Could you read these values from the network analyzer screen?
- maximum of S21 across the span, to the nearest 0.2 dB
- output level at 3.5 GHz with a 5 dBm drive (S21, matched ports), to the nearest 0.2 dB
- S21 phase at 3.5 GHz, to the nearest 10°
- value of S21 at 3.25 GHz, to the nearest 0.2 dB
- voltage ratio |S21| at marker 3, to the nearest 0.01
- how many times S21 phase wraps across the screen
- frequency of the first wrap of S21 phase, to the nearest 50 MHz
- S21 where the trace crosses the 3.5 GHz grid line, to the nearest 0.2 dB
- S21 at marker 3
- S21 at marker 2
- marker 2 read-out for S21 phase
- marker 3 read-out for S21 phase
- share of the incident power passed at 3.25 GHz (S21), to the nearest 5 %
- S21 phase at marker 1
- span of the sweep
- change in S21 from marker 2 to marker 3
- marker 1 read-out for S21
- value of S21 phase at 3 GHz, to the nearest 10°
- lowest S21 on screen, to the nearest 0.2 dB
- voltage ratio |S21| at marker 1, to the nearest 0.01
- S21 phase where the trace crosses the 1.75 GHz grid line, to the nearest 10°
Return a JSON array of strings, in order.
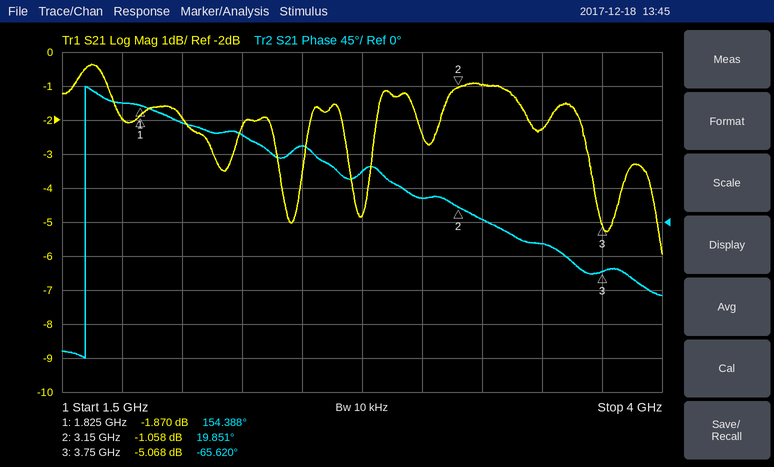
["-0.4 dB", "2.8 dBm", "-30°", "-1.0 dB", "0.56", "1", "1.60 GHz", "-2.2 dB", "-5.068 dB", "-1.058 dB", "19.851°", "-65.620°", "80 %", "154.388°", "2.5 GHz", "-4.010 dB", "-1.870 dB", "30°", "-6.0 dB", "0.81", "160°"]
